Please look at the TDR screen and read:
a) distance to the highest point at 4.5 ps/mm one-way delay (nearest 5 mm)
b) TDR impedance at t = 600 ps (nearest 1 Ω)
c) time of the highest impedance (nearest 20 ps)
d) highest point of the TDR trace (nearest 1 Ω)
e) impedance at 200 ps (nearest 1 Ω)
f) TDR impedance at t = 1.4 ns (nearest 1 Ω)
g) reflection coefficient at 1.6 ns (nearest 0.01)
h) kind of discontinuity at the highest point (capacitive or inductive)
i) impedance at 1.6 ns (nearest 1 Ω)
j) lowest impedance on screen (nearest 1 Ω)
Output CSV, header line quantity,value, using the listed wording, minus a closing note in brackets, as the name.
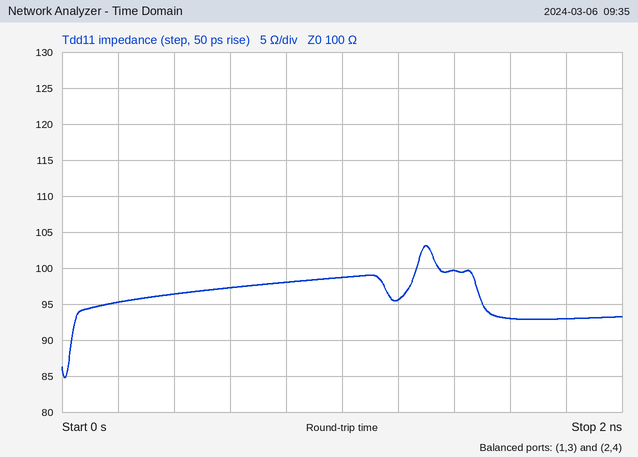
quantity,value
distance to the highest point at 4.5 ps/mm one-way delay,145 mm
TDR impedance at t = 600 ps,97 Ω
time of the highest impedance,1.30 ns
highest point of the TDR trace,103 Ω
impedance at 200 ps,95 Ω
TDR impedance at t = 1.4 ns,100 Ω
reflection coefficient at 1.6 ns,-0.04
kind of discontinuity at the highest point,inductive
impedance at 1.6 ns,93 Ω
lowest impedance on screen,85 Ω
